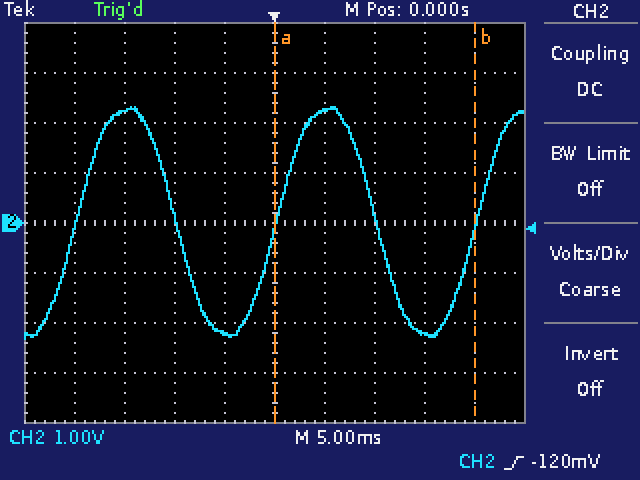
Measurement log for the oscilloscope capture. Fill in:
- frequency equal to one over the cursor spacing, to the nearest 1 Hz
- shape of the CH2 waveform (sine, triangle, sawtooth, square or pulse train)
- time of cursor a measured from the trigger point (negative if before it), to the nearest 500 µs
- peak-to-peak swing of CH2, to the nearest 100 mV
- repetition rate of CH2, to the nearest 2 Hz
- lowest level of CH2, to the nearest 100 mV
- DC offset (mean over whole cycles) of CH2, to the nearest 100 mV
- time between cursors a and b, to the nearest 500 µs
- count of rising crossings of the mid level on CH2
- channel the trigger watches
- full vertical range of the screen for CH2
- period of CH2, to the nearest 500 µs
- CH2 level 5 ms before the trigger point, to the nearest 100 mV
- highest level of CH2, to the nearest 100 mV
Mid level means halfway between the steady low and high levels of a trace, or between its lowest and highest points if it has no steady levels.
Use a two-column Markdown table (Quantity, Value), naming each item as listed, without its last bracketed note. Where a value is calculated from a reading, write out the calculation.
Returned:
| Quantity | Value |
|---|---|
| frequency equal to one over the cursor spacing, to the nearest 1 Hz | 1 / 20.0 ms ≈ 50 Hz |
| shape of the CH2 waveform | sine |
| time of cursor a measured from the trigger point (negative if before it), to the nearest 500 µs | 0.0 ms |
| peak-to-peak swing of CH2, to the nearest 100 mV | 2.3 V − (-2.3 V) = 4.6 V |
| repetition rate of CH2, to the nearest 2 Hz | 1 / 20.0 ms ≈ 50 Hz |
| lowest level of CH2, to the nearest 100 mV | -2.3 V |
| DC offset (mean over whole cycles) of CH2, to the nearest 100 mV | (2.3 V + (-2.3 V)) / 2 ≈ 0.0 V |
| time between cursors a and b, to the nearest 500 µs | 20.0 ms |
| count of rising crossings of the mid level on CH2 | 3 |
| channel the trigger watches | CH2 |
| full vertical range of the screen for CH2 | 8 V |
| period of CH2, to the nearest 500 µs | 20.0 ms |
| CH2 level 5 ms before the trigger point, to the nearest 100 mV | -2.2 V |
| highest level of CH2, to the nearest 100 mV | 2.3 V |
